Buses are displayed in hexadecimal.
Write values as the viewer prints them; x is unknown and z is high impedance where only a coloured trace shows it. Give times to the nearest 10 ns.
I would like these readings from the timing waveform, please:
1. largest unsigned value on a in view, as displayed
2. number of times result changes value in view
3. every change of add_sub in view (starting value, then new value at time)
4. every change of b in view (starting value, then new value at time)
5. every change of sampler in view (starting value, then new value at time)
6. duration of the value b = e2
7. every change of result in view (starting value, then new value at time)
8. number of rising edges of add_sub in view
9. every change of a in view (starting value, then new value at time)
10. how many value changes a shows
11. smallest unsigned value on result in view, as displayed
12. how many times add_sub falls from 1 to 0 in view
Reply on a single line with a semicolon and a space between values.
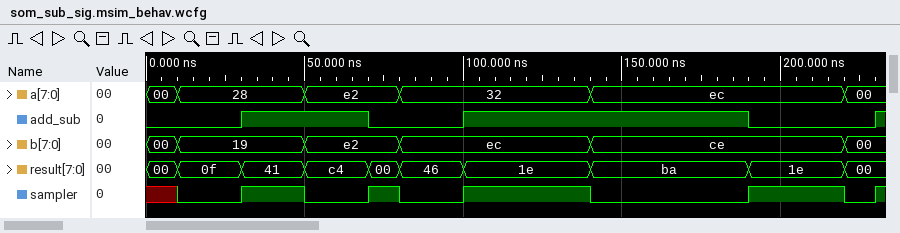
ec; 9; 0, 1 at 30 ns, 0 at 70 ns, 1 at 100 ns, 0 at 190 ns, 1 at 230 ns; 00, 19 at 10 ns, e2 at 50 ns, ec at 80 ns, ce at 140 ns, 00 at 220 ns; x, 0 at 10 ns, 1 at 30 ns, 0 at 50 ns, 1 at 70 ns, 0 at 80 ns, 1 at 100 ns, 0 at 140 ns, 1 at 190 ns, 0 at 220 ns, 1 at 230 ns; 30 ns; 00, 0f at 10 ns, 41 at 30 ns, c4 at 50 ns, 00 at 70 ns, 46 at 80 ns, 1e at 100 ns, ba at 140 ns, 1e at 190 ns, 00 at 220 ns; 3; 00, 28 at 10 ns, e2 at 50 ns, 32 at 80 ns, ec at 140 ns, 00 at 220 ns; 5; 00; 2
